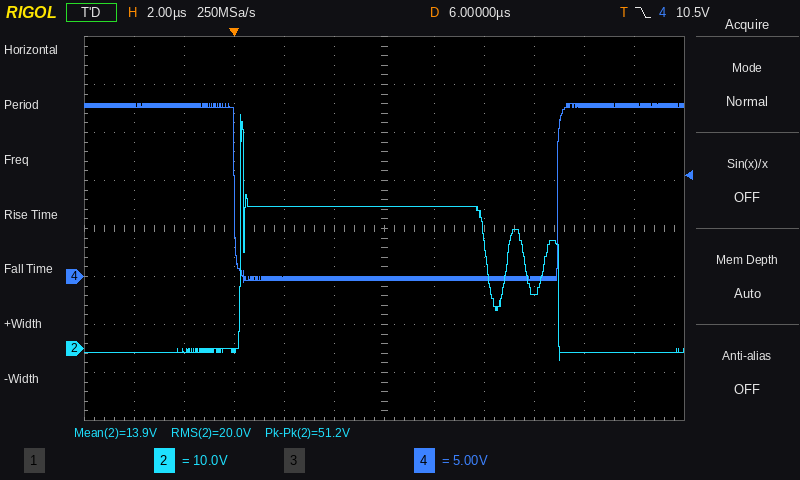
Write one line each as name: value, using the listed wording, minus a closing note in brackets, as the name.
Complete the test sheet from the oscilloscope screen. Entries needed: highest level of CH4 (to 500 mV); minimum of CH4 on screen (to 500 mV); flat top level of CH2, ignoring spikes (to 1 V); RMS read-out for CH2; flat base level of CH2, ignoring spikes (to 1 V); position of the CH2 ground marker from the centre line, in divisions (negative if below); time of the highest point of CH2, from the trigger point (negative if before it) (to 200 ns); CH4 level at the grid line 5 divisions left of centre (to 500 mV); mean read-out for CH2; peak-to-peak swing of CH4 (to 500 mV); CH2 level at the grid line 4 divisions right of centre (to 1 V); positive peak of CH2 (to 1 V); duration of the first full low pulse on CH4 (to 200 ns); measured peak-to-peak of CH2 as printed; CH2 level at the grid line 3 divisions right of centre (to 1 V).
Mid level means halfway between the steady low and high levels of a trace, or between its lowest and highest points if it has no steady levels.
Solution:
highest level of CH4: 18.0 V
minimum of CH4 on screen: -500 mV
flat top level of CH2, ignoring spikes: 30 V
RMS read-out for CH2: 20.0 V
flat base level of CH2, ignoring spikes: -1 V
position of the CH2 ground marker from the centre line, in divisions: -2.5 div
time of the highest point of CH2, from the trigger point (negative if before it): +200 ns
CH4 level at the grid line 5 divisions left of centre: 18.0 V
mean read-out for CH2: 13.9 V
peak-to-peak swing of CH4: 18.5 V
CH2 level at the grid line 4 divisions right of centre: -1 V
positive peak of CH2: 49 V
duration of the first full low pulse on CH4: 13.0 µs
measured peak-to-peak of CH2 as printed: 51.2 V
CH2 level at the grid line 3 divisions right of centre: 11 V
